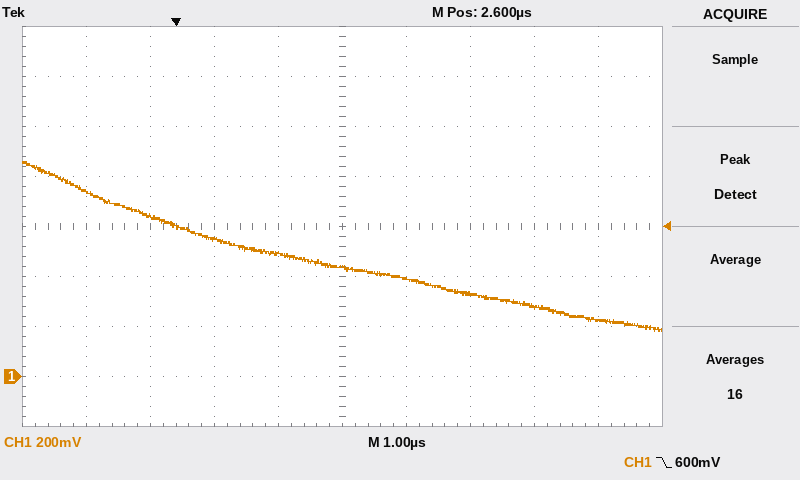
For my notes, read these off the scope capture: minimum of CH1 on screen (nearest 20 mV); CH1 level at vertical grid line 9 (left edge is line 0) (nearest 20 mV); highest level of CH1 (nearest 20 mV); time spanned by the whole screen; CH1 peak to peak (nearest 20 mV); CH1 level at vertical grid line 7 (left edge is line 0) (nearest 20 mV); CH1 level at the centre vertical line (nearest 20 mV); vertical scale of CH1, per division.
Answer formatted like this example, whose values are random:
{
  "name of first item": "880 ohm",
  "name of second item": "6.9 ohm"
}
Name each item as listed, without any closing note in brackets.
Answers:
{
  "minimum of CH1 on screen": "180 mV",
  "CH1 level at vertical grid line 9 (left edge is line 0)": "220 mV",
  "highest level of CH1": "860 mV",
  "time spanned by the whole screen": "10 µs",
  "CH1 peak to peak": "680 mV",
  "CH1 level at vertical grid line 7 (left edge is line 0)": "340 mV",
  "CH1 level at the centre vertical line": "440 mV",
  "vertical scale of CH1, per division": "200 mV"
}
